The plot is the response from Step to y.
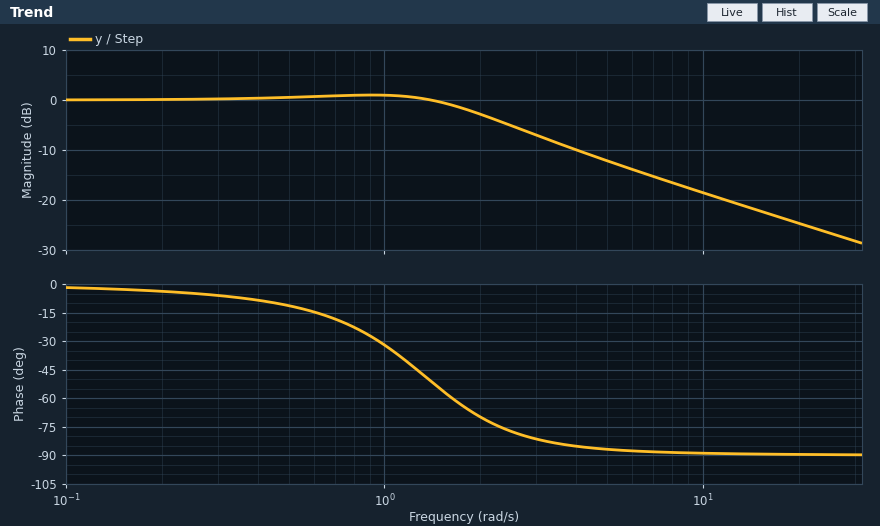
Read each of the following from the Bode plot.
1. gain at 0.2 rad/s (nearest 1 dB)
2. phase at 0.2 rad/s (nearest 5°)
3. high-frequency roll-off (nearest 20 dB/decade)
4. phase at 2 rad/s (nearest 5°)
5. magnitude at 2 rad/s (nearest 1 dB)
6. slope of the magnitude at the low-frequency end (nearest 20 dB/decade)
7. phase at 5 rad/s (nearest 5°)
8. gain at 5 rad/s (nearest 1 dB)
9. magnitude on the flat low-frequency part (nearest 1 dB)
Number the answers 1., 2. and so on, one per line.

1. 0 dB
2. -5°
3. -20 dB/decade
4. -70°
5. -3 dB
6. 0 dB/decade
7. -85°
8. -12 dB
9. 0 dB
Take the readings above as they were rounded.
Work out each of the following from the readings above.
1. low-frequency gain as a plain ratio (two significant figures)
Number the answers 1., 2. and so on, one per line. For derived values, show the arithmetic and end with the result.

1. 10^(0 / 20) = 1.0
